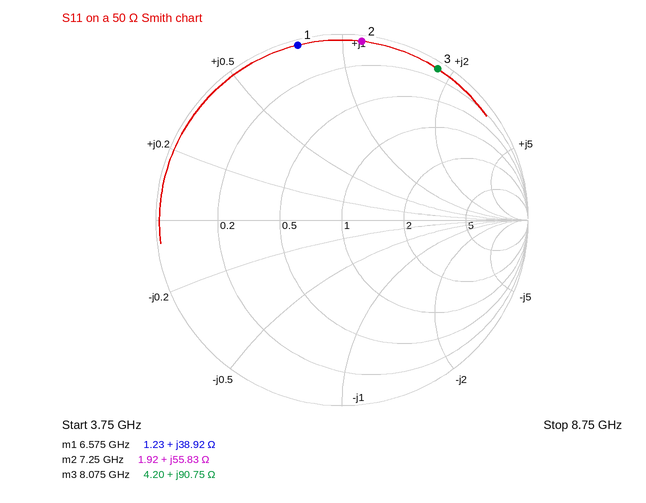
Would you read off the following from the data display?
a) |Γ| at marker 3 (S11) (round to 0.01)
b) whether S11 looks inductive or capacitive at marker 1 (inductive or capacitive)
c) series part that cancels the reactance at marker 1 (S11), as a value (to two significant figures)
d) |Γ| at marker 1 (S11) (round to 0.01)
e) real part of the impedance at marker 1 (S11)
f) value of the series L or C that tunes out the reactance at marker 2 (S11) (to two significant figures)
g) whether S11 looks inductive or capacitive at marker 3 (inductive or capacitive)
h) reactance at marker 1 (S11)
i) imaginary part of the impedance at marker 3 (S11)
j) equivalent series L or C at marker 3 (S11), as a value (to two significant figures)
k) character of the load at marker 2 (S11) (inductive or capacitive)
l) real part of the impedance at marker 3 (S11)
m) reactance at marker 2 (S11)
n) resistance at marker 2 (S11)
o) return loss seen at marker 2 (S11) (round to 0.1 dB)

0.96
inductive
620 fF
0.97
1.23 Ω
390 fF
inductive
+38.92 Ω
+90.75 Ω
1.8 nH
inductive
4.20 Ω
+55.83 Ω
1.92 Ω
0.3 dB
